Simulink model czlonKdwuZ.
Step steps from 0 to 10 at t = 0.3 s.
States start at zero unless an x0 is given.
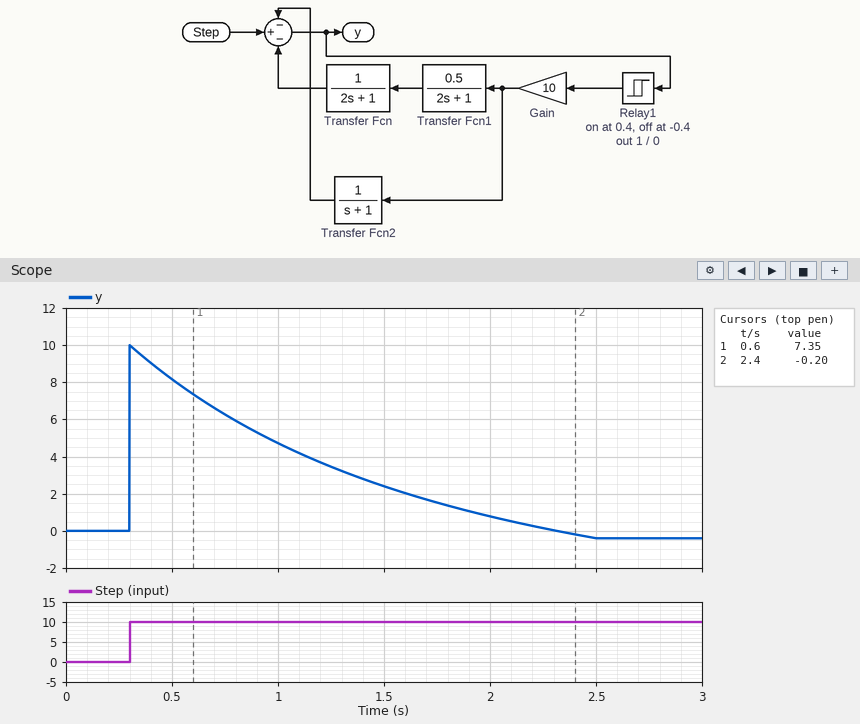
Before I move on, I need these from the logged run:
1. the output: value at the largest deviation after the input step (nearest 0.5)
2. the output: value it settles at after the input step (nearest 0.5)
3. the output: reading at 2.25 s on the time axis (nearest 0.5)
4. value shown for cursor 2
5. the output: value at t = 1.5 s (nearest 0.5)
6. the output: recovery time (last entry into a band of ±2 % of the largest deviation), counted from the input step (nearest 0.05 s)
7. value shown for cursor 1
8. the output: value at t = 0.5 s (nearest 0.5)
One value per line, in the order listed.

10.0
-0.5
0.0
-0.20
2.5
2.10 s
7.35
8.0
